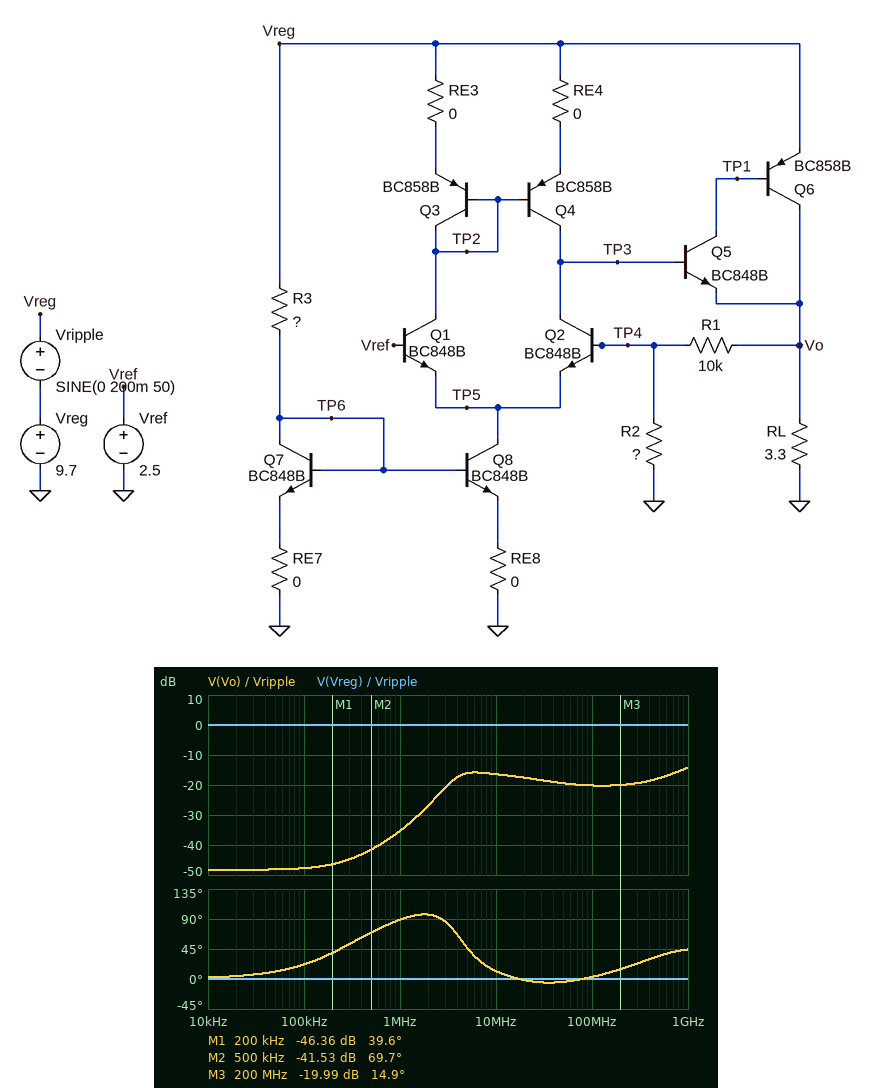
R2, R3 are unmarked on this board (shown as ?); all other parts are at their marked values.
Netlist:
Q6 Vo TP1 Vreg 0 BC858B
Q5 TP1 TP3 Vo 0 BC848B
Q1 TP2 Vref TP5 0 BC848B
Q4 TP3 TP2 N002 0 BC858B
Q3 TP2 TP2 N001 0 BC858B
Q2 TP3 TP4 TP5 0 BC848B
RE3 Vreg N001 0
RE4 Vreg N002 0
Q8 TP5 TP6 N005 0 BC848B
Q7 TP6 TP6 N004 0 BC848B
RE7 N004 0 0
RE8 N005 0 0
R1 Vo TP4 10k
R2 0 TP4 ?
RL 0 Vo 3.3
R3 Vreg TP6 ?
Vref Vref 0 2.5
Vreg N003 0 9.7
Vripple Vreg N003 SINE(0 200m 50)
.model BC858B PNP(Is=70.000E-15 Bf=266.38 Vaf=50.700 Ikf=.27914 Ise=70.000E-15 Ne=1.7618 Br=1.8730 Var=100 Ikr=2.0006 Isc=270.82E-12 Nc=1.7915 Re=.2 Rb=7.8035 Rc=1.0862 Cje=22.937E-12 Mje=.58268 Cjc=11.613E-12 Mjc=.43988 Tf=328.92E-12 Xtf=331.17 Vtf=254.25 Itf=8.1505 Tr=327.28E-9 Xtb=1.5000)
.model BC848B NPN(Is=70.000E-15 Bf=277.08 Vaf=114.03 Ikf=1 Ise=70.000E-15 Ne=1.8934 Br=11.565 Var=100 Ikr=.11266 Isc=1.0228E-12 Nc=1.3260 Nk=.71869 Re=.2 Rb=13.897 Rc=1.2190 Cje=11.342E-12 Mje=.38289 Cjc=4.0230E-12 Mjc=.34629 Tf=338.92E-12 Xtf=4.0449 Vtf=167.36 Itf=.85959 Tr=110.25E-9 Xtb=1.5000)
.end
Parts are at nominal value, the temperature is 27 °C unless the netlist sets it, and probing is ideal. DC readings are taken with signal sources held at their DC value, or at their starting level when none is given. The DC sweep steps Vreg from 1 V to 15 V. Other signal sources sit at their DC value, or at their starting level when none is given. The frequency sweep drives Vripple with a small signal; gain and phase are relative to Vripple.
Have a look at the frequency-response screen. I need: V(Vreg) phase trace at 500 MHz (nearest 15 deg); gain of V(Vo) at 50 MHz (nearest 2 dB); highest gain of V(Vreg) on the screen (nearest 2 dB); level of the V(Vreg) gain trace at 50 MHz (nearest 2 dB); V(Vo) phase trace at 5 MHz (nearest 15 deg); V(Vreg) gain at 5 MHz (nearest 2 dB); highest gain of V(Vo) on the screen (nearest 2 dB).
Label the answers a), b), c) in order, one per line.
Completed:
a) 0 deg
b) -20 dB
c) 0 dB
d) 0 dB
e) 45 deg
f) 0 dB
g) -14 dB
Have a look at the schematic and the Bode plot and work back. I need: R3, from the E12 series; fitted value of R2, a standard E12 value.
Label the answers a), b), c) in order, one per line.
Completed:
a) 10 kΩ
b) 22 kΩ
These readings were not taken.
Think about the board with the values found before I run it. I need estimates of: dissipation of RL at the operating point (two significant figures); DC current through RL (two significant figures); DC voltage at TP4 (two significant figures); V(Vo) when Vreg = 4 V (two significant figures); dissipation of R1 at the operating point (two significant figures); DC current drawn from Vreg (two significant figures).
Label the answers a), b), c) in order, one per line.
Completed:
a) 4.0 W
b) 1.1 A
c) 2.5 V
d) 2.8 V
e) 130 µW
f) 1.1 A
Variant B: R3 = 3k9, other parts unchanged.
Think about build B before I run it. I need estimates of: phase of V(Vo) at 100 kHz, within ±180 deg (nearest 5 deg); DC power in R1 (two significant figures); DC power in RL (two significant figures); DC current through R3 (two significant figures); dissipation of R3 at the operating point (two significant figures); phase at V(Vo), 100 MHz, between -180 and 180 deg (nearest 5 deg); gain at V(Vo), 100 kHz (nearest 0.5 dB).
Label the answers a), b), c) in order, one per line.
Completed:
a) 10 deg
b) 140 µW
c) 4.1 W
d) 2.3 mA
e) 21 mW
f) 0 deg
g) -43.5 dB
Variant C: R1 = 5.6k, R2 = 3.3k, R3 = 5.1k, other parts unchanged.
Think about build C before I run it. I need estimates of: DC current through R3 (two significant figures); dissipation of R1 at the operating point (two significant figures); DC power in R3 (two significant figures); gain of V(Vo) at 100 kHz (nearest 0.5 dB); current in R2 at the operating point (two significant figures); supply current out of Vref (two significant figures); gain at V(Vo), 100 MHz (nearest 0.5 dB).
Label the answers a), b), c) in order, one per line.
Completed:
a) 1.8 mA
b) 3.2 mW
c) 16 mW
d) -42.0 dB
e) 760 µA
f) 3.5 µA
g) -15.0 dB
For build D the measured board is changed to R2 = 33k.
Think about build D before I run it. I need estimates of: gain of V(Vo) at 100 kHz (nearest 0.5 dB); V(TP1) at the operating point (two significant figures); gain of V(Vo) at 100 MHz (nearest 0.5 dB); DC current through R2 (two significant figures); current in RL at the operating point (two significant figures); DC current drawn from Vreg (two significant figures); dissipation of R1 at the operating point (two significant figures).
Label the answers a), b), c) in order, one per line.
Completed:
a) -48.5 dB
b) 8.6 V
c) -20.5 dB
d) 76 µA
e) 990 mA
f) 1.0 A
g) 60 µW
